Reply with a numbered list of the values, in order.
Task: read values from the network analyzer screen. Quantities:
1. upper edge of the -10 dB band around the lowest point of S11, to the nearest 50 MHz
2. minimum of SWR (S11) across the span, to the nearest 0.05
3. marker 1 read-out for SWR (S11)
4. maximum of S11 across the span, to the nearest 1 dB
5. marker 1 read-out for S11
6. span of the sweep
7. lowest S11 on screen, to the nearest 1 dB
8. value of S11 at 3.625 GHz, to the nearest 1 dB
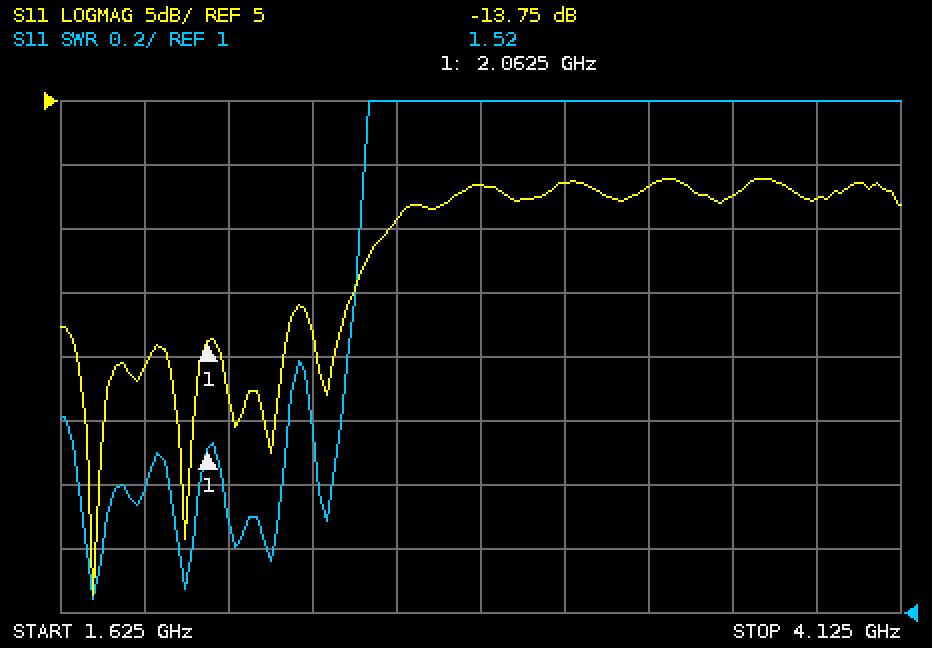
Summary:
1. 2.50 GHz
2. 1.05
3. 1.52
4. -1 dB
5. -13.75 dB
6. 2.5 GHz
7. -34 dB
8. -2 dB
